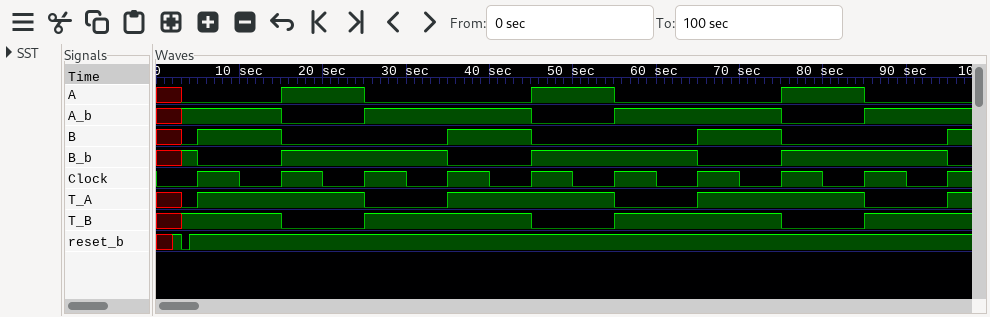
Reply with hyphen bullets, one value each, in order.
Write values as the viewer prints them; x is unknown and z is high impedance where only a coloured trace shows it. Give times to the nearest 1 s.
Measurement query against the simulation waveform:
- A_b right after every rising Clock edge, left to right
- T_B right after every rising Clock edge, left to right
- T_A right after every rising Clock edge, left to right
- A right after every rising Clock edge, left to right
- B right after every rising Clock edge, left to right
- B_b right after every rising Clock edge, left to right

- 1 0 1 1 0 1 1 0 1 1
- 1 0 1 1 0 1 1 0 1 1
- 1 1 0 1 1 0 1 1 0 1
- 0 1 0 0 1 0 0 1 0 0
- 1 0 0 1 0 0 1 0 0 1
- 0 1 1 0 1 1 0 1 1 0
